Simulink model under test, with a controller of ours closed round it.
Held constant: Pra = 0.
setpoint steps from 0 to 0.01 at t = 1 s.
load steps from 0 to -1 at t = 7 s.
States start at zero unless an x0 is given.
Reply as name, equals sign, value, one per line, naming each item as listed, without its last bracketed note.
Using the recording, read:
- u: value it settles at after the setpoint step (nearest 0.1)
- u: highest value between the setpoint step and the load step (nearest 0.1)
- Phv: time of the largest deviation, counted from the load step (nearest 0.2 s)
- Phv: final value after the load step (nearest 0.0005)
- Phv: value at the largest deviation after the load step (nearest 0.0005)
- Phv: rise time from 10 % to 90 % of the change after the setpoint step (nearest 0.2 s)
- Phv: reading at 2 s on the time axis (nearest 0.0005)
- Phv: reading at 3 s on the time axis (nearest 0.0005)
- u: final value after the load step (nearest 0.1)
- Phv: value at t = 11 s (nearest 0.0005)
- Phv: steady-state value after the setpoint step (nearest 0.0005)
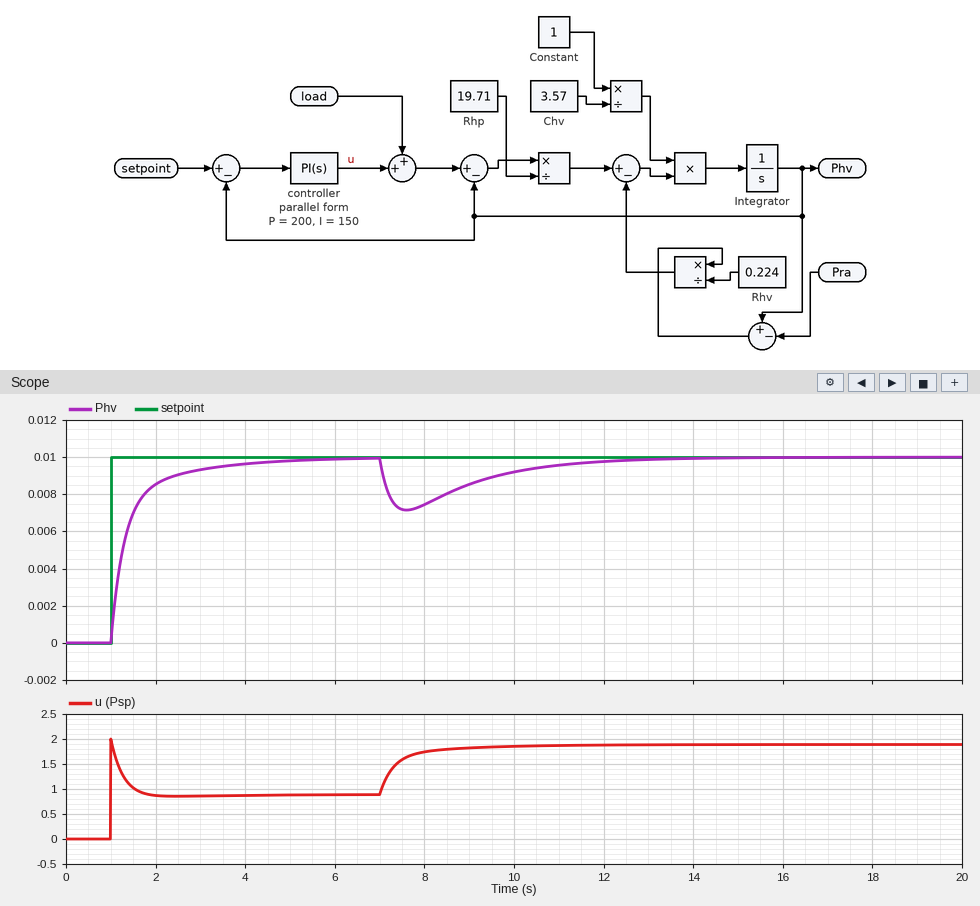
u: value it settles at after the setpoint step = 0.9
u: highest value between the setpoint step and the load step = 2.0
Phv: time of the largest deviation, counted from the load step = 0.6 s
Phv: final value after the load step = 0.0100
Phv: value at the largest deviation after the load step = 0.0070
Phv: rise time from 10 % to 90 % of the change after the setpoint step = 1.4 s
Phv: reading at 2 s on the time axis = 0.0085
Phv: reading at 3 s on the time axis = 0.0095
u: final value after the load step = 1.9
Phv: value at t = 11 s = 0.0095
Phv: steady-state value after the setpoint step = 0.0100
